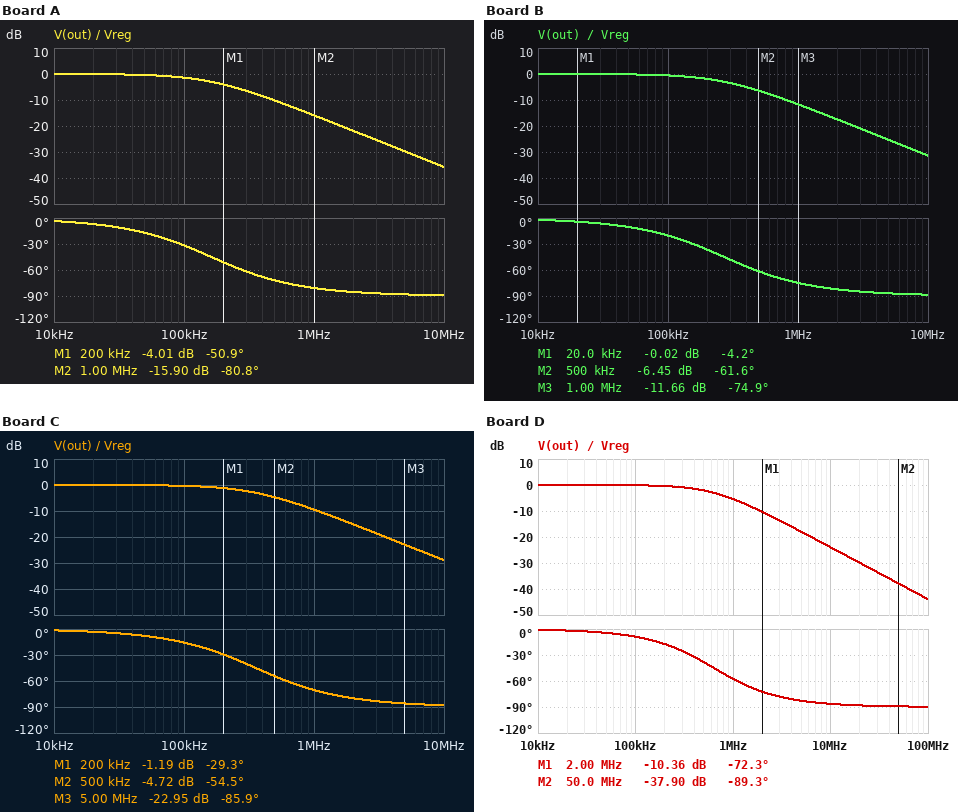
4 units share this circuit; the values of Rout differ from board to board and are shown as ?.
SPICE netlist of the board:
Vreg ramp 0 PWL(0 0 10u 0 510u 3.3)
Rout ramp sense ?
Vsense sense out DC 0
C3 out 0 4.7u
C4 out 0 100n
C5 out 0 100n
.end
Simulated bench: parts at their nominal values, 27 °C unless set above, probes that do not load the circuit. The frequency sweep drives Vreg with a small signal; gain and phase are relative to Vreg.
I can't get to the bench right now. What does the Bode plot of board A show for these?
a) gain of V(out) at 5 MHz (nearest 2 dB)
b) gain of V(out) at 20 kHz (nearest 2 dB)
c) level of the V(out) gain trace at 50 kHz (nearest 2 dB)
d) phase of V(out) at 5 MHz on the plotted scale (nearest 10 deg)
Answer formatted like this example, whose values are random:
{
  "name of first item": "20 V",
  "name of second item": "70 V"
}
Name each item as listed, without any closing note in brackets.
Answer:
{
  "gain of V(out) at 5 MHz": "-30 dB",
  "gain of V(out) at 20 kHz": "0 dB",
  "level of the V(out) gain trace at 50 kHz": "0 dB",
  "phase of V(out) at 5 MHz on the plotted scale": "-90 deg"
}
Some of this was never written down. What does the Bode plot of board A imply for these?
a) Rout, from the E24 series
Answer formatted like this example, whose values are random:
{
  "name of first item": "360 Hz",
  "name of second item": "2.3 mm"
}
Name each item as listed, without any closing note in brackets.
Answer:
{
  "Rout, from the E24 series": "0.2 Ω"
}
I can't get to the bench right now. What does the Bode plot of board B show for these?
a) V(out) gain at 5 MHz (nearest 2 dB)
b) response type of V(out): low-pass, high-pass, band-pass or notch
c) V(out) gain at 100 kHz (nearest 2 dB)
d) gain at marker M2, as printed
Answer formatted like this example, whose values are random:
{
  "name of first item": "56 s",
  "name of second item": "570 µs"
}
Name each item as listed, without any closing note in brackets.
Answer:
{
  "V(out) gain at 5 MHz": "-26 dB",
  "response type of V(out): low-pass, high-pass, band-pass or notch": "low-pass",
  "V(out) gain at 100 kHz": "0 dB",
  "gain at marker M2, as printed": "-6.45 dB"
}
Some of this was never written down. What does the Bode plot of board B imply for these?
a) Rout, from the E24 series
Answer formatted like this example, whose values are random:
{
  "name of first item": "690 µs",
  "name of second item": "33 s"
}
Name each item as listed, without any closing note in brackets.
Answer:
{
  "Rout, from the E24 series": "0.12 Ω"
}
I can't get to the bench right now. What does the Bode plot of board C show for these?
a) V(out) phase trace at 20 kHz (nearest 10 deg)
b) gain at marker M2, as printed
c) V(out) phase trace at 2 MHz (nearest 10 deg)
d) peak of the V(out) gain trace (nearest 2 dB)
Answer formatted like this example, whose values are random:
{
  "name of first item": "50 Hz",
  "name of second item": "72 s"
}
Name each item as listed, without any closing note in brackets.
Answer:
{
  "V(out) phase trace at 20 kHz": "0 deg",
  "gain at marker M2, as printed": "-4.72 dB",
  "V(out) phase trace at 2 MHz": "-80 deg",
  "peak of the V(out) gain trace": "0 dB"
}
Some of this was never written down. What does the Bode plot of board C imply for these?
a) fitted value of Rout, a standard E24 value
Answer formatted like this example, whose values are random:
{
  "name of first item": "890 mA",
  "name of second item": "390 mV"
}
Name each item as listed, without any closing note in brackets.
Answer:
{
  "fitted value of Rout, a standard E24 value": "0.091 Ω"
}
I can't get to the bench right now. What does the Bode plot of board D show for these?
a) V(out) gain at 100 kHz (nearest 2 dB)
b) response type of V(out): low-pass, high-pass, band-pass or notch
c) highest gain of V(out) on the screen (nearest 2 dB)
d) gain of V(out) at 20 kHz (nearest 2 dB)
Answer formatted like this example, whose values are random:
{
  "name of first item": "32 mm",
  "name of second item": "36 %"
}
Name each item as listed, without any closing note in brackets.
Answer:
{
  "V(out) gain at 100 kHz": "0 dB",
  "response type of V(out): low-pass, high-pass, band-pass or notch": "low-pass",
  "highest gain of V(out) on the screen": "0 dB",
  "gain of V(out) at 20 kHz": "0 dB"
}
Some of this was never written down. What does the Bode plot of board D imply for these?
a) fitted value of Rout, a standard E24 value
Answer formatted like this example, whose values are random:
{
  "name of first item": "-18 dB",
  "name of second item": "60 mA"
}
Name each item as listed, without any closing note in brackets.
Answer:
{
  "fitted value of Rout, a standard E24 value": "0.051 Ω"
}
